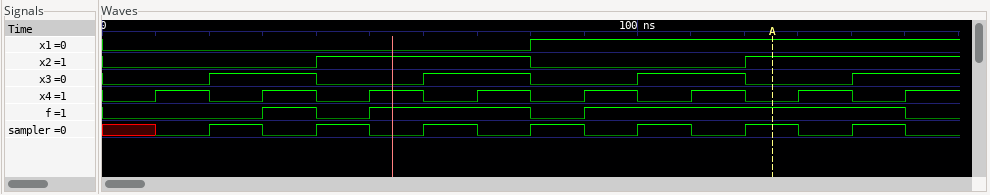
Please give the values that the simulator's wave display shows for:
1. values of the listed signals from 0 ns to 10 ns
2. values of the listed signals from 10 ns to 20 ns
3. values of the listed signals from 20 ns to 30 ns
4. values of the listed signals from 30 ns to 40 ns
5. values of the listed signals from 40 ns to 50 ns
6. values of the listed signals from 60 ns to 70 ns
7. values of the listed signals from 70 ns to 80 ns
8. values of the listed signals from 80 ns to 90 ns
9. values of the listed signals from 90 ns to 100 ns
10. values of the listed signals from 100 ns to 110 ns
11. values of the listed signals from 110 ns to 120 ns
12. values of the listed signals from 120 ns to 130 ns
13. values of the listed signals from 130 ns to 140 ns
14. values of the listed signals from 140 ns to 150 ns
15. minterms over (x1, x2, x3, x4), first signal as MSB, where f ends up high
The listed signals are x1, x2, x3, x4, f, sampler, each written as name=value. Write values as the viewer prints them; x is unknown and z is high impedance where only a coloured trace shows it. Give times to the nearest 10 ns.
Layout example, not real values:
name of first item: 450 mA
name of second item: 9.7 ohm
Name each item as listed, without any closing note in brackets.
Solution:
values of the listed signals from 0 ns to 10 ns: x1=0, x2=0, x3=0, x4=0, f=0, sampler=x
values of the listed signals from 10 ns to 20 ns: x1=0, x2=0, x3=0, x4=1, f=0, sampler=0
values of the listed signals from 20 ns to 30 ns: x1=0, x2=0, x3=1, x4=0, f=0, sampler=1
values of the listed signals from 30 ns to 40 ns: x1=0, x2=0, x3=1, x4=1, f=1, sampler=0
values of the listed signals from 40 ns to 50 ns: x1=0, x2=1, x3=0, x4=0, f=0, sampler=1
values of the listed signals from 60 ns to 70 ns: x1=0, x2=1, x3=1, x4=0, f=1, sampler=1
values of the listed signals from 70 ns to 80 ns: x1=0, x2=1, x3=1, x4=1, f=1, sampler=0
values of the listed signals from 80 ns to 90 ns: x1=1, x2=0, x3=0, x4=0, f=0, sampler=1
values of the listed signals from 90 ns to 100 ns: x1=1, x2=0, x3=0, x4=1, f=1, sampler=0
values of the listed signals from 100 ns to 110 ns: x1=1, x2=0, x3=1, x4=0, f=1, sampler=1
values of the listed signals from 110 ns to 120 ns: x1=1, x2=0, x3=1, x4=1, f=1, sampler=0
values of the listed signals from 120 ns to 130 ns: x1=1, x2=1, x3=0, x4=0, f=1, sampler=1
values of the listed signals from 130 ns to 140 ns: x1=1, x2=1, x3=0, x4=1, f=1, sampler=0
values of the listed signals from 140 ns to 150 ns: x1=1, x2=1, x3=1, x4=0, f=1, sampler=1
minterms over (x1, x2, x3, x4), first signal as MSB, where f ends up high: 3, 5, 6, 7, 9, 10, 11, 12, 13, 14
